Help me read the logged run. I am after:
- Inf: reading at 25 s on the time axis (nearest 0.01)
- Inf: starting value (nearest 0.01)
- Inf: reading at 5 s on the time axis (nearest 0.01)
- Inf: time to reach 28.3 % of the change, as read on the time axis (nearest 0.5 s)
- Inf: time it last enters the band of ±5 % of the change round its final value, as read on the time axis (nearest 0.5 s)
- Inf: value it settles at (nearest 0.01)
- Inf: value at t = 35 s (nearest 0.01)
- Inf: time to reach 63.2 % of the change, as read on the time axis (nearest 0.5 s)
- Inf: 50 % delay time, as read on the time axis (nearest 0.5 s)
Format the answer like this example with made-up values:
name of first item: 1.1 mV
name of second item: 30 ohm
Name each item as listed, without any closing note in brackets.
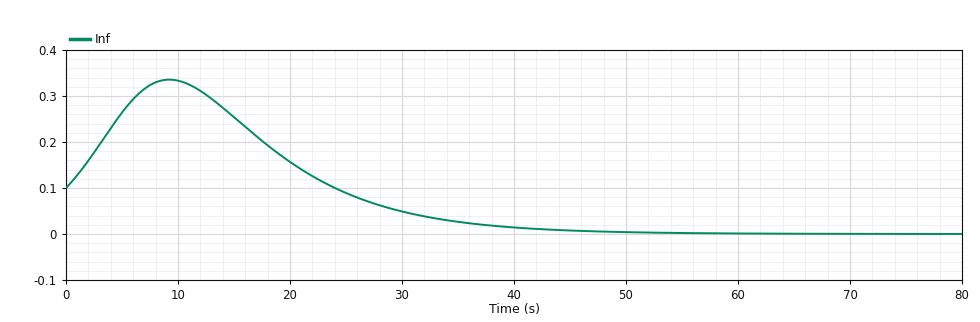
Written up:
Inf: reading at 25 s on the time axis: 0.09
Inf: starting value: 0.10
Inf: reading at 5 s on the time axis: 0.26
Inf: time to reach 28.3 % of the change, as read on the time axis: 27.0 s
Inf: time it last enters the band of ±5 % of the change round its final value, as read on the time axis: 48.5 s
Inf: value it settles at: 0.00
Inf: value at t = 35 s: 0.03
Inf: time to reach 63.2 % of the change, as read on the time axis: 32.5 s
Inf: 50 % delay time, as read on the time axis: 30.0 s
